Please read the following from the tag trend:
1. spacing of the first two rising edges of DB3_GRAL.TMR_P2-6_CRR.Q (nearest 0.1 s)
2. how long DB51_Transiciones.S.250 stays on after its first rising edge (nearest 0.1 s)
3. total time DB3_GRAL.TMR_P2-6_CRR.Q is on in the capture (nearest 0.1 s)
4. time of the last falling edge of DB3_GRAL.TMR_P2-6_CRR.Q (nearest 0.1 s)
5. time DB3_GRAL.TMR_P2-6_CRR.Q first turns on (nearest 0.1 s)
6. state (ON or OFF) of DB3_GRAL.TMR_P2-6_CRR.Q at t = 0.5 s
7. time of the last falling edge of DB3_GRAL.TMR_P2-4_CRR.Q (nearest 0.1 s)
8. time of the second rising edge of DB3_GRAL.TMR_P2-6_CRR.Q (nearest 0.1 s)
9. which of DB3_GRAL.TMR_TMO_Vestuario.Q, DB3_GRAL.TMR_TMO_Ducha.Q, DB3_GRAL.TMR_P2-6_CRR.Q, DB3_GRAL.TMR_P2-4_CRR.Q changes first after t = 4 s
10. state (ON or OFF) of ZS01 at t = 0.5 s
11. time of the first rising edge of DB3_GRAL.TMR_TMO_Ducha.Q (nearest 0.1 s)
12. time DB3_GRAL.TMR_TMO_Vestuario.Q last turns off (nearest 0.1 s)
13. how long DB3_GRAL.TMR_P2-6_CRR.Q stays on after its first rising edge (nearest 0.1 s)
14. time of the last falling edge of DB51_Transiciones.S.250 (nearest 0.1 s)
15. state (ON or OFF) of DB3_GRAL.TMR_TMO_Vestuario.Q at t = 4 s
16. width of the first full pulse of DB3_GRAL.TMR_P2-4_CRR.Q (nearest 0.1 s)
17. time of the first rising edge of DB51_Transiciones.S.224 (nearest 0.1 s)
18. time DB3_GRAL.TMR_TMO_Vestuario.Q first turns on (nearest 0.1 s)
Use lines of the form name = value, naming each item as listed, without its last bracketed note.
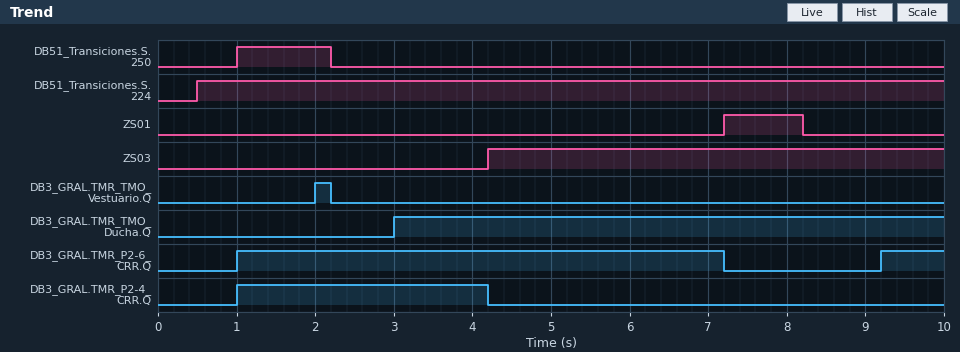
spacing of the first two rising edges of DB3_GRAL.TMR_P2-6_CRR.Q = 8.2 s
how long DB51_Transiciones.S.250 stays on after its first rising edge = 1.2 s
total time DB3_GRAL.TMR_P2-6_CRR.Q is on in the capture = 7.0 s
time of the last falling edge of DB3_GRAL.TMR_P2-6_CRR.Q = 7.2 s
time DB3_GRAL.TMR_P2-6_CRR.Q first turns on = 1.0 s
state (ON or OFF) of DB3_GRAL.TMR_P2-6_CRR.Q at t = 0.5 s = OFF
time of the last falling edge of DB3_GRAL.TMR_P2-4_CRR.Q = 4.2 s
time of the second rising edge of DB3_GRAL.TMR_P2-6_CRR.Q = 9.2 s
which of DB3_GRAL.TMR_TMO_Vestuario.Q, DB3_GRAL.TMR_TMO_Ducha.Q, DB3_GRAL.TMR_P2-6_CRR.Q, DB3_GRAL.TMR_P2-4_CRR.Q changes first after t = 4 s = DB3_GRAL.TMR_P2-4_CRR.Q
state (ON or OFF) of ZS01 at t = 0.5 s = OFF
time of the first rising edge of DB3_GRAL.TMR_TMO_Ducha.Q = 3.0 s
time DB3_GRAL.TMR_TMO_Vestuario.Q last turns off = 2.2 s
how long DB3_GRAL.TMR_P2-6_CRR.Q stays on after its first rising edge = 6.2 s
time of the last falling edge of DB51_Transiciones.S.250 = 2.2 s
state (ON or OFF) of DB3_GRAL.TMR_TMO_Vestuario.Q at t = 4 s = OFF
width of the first full pulse of DB3_GRAL.TMR_P2-4_CRR.Q = 3.2 s
time of the first rising edge of DB51_Transiciones.S.224 = 0.5 s
time DB3_GRAL.TMR_TMO_Vestuario.Q first turns on = 2.0 s
